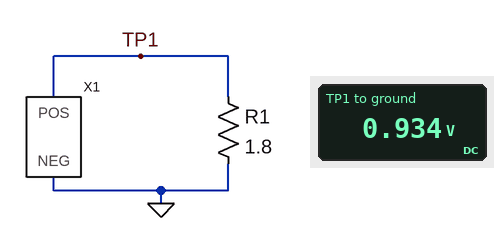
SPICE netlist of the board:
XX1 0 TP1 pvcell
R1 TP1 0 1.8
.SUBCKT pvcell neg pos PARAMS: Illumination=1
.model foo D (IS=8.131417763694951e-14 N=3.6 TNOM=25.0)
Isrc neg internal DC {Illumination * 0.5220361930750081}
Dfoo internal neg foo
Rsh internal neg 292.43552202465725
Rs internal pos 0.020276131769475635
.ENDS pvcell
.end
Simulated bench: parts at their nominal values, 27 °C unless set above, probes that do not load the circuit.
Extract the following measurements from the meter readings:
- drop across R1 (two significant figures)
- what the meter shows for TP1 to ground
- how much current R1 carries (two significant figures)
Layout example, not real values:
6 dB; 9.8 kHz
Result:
930 mV; 0.934 V; 520 mA
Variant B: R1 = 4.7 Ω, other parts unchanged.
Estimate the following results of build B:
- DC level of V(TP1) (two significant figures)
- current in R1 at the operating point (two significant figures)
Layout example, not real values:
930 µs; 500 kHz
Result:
2.4 V; 500 mA
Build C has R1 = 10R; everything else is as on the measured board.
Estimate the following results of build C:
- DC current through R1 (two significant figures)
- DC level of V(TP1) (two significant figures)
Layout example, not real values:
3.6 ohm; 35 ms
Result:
270 mA; 2.7 V
